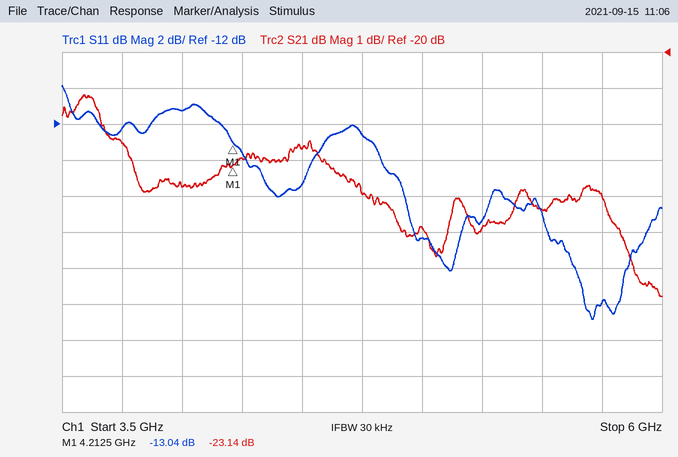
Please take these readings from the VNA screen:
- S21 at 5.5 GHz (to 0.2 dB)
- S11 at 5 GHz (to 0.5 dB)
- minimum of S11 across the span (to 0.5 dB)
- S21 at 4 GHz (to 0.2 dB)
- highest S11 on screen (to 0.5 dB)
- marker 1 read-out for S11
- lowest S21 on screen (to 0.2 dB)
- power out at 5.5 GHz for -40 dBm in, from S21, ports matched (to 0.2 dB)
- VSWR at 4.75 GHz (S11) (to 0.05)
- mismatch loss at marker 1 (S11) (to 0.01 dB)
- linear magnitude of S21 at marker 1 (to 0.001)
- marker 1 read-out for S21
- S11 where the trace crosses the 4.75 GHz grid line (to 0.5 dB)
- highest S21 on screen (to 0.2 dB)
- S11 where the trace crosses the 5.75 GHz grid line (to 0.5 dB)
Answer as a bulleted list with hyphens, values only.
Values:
- -24.4 dB
- -18.5 dB
- -23.0 dB
- -23.8 dB
- -10.0 dB
- -13.04 dB
- -26.8 dB
- -64.4 dBm
- 1.60
- 0.22 dB
- 0.070
- -23.14 dB
- -12.5 dB
- -21.2 dB
- -22.0 dB
